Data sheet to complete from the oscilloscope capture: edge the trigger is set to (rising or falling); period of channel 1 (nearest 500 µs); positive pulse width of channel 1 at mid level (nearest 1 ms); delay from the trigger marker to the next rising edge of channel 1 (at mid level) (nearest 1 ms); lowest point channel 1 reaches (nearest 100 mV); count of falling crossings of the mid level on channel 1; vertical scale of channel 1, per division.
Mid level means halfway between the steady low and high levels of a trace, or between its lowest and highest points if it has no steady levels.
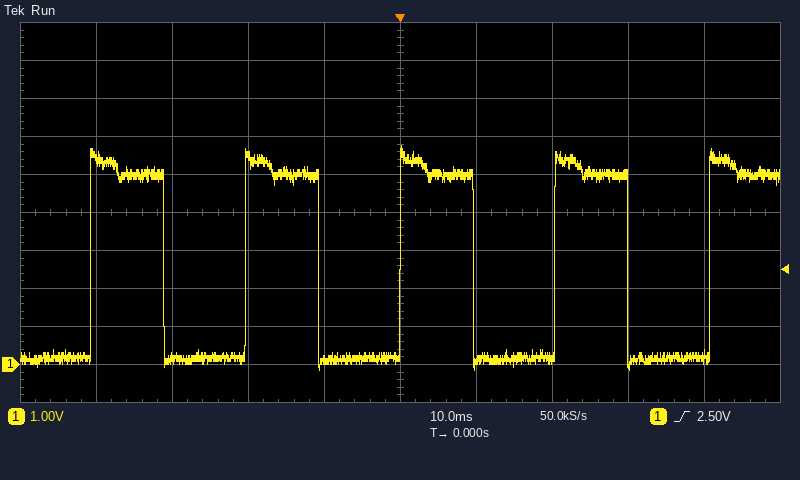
rising
20.5 ms
10 ms
20 ms
-200 mV
4
1 V
